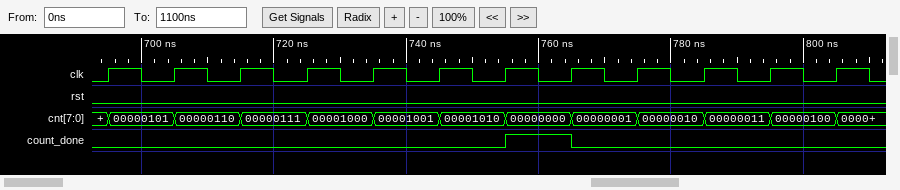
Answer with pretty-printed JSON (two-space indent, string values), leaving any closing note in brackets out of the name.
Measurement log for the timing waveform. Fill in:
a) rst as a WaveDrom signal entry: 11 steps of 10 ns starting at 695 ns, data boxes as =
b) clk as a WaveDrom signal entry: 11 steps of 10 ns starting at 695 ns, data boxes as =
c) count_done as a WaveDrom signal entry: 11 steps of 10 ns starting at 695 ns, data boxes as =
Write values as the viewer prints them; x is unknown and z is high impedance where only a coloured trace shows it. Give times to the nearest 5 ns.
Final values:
{
  "rst as a WaveDrom signal entry: 11 steps of 10 ns starting at 695 ns, data boxes as =": "{name: 'rst', wave: '0..........'}",
  "clk as a WaveDrom signal entry: 11 steps of 10 ns starting at 695 ns, data boxes as =": "{name: 'clk', wave: 'p..........'}",
  "count_done as a WaveDrom signal entry: 11 steps of 10 ns starting at 695 ns, data boxes as =": "{name: 'count_done', wave: '0.....10...'}"
}
